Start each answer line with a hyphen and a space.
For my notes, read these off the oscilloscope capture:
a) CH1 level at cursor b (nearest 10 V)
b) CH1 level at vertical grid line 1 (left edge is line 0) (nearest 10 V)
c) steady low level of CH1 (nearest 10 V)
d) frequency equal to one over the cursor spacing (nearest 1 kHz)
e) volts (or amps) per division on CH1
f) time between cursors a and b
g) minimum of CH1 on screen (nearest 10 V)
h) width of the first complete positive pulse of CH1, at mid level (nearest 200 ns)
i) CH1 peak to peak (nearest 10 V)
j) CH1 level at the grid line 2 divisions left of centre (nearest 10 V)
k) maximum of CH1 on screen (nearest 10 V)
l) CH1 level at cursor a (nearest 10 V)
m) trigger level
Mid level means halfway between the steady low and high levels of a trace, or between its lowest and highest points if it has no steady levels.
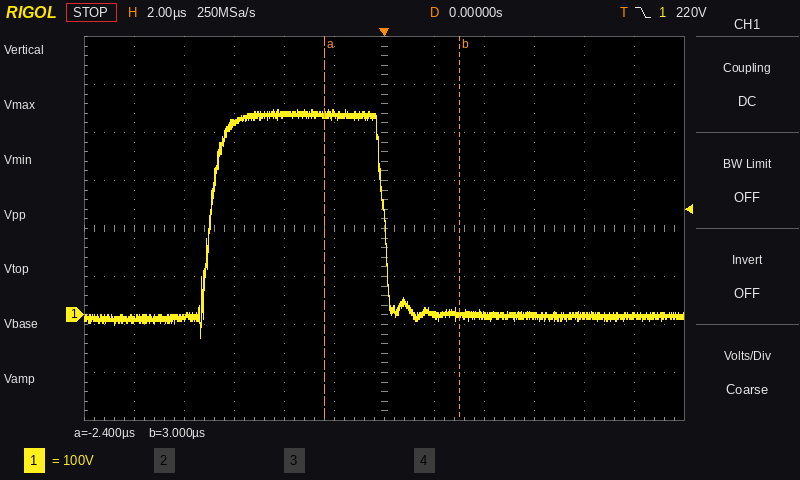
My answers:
- 0 V
- -10 V
- 0 V
- 185 kHz
- 100 V
- 5.4 µs
- -50 V
- 7.0 µs
- 480 V
- 420 V
- 430 V
- 420 V
- 220 V
